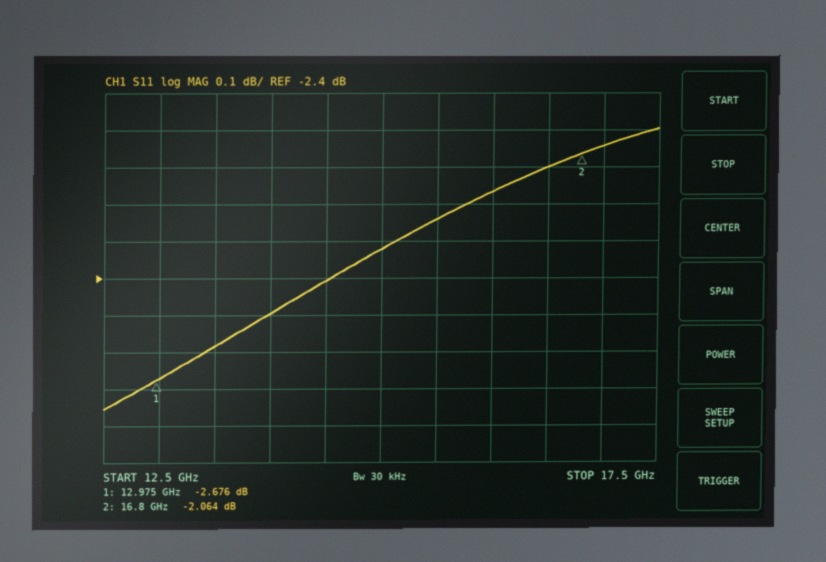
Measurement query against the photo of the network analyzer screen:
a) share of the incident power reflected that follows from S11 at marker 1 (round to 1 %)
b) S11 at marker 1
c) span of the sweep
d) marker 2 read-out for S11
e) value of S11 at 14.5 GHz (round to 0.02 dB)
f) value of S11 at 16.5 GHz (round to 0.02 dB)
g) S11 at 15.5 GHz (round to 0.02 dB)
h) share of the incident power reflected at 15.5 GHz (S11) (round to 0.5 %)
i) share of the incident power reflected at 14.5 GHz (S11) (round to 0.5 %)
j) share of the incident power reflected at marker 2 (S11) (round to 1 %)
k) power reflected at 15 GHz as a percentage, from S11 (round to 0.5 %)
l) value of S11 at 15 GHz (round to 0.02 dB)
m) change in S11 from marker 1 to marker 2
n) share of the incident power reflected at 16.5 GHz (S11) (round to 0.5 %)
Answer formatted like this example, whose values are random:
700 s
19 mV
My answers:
54 %
-2.676 dB
5 GHz
-2.064 dB
-2.40 dB
-2.10 dB
-2.24 dB
59.5 %
57.5 %
62 %
58.5 %
-2.32 dB
0.612 dB
61.5 %
